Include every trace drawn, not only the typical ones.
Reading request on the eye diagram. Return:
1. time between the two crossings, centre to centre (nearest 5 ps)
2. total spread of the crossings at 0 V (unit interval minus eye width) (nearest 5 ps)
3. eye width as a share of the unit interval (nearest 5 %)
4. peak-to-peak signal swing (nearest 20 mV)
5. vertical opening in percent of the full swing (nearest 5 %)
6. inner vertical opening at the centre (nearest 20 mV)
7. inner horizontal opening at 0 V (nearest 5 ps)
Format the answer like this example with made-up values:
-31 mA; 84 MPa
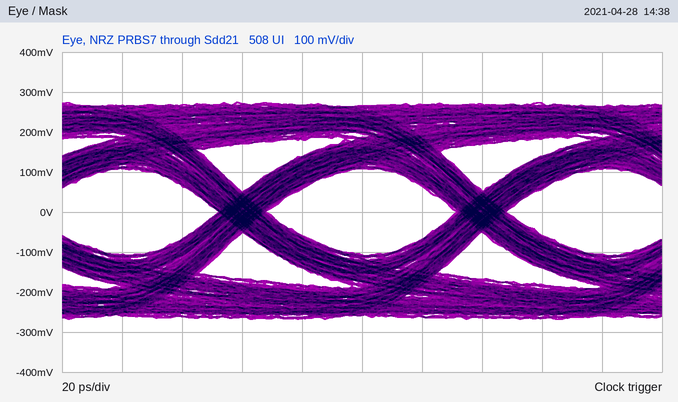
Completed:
80 ps; 15 ps; 80 %; 540 mV; 40 %; 220 mV; 65 ps
